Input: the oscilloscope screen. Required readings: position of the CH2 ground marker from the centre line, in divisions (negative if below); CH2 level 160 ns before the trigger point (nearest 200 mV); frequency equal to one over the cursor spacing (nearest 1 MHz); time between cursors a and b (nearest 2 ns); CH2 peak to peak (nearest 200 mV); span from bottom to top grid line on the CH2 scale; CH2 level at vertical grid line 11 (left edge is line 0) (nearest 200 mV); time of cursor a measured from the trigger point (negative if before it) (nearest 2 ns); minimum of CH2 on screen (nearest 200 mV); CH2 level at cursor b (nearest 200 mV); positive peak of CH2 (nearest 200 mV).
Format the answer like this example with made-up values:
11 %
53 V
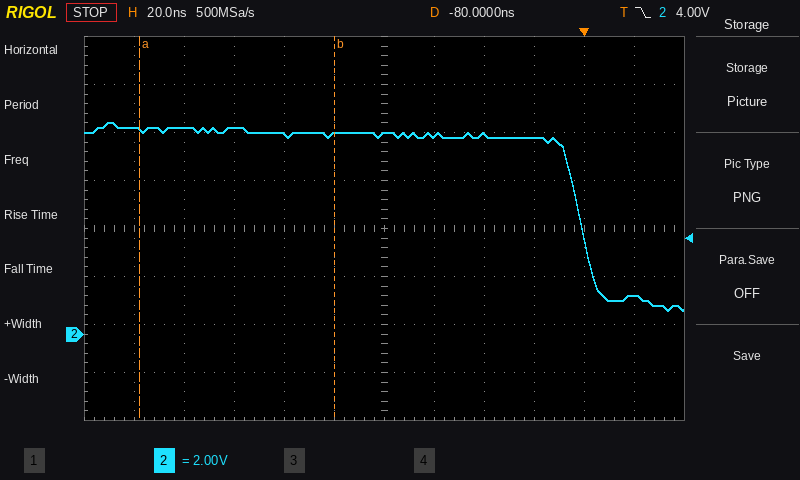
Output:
-2.2 div
8.6 V
13 MHz
78 ns
7.8 V
16 V
1.6 V
-178 ns
1.0 V
8.4 V
8.8 V
